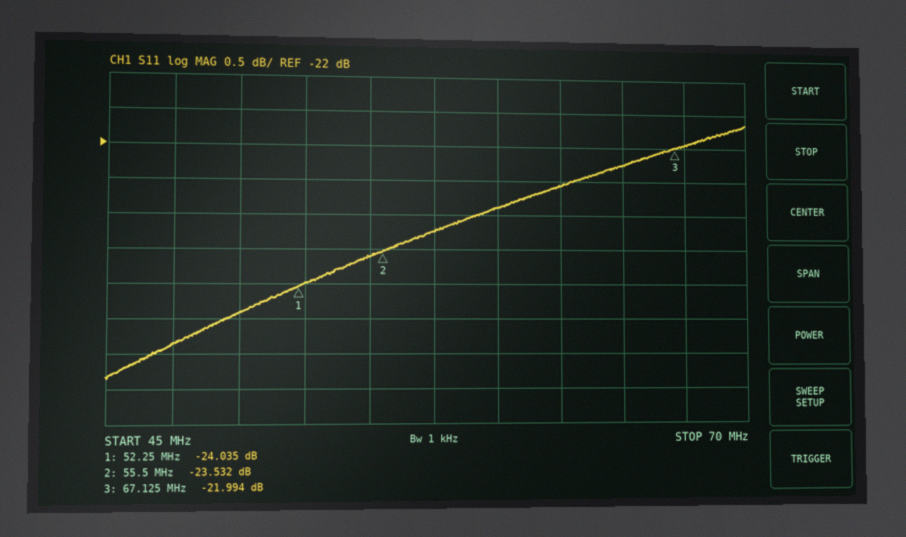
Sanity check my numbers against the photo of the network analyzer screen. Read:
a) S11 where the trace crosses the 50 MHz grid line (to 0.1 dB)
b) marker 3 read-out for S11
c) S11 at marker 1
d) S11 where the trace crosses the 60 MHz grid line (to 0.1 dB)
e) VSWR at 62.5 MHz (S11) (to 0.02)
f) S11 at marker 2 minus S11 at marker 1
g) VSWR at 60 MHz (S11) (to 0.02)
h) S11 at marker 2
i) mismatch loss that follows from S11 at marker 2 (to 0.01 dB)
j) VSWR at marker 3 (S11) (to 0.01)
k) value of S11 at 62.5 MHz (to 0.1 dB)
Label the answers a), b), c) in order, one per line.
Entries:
a) -24.4 dB
b) -21.994 dB
c) -24.035 dB
d) -22.9 dB
e) 1.16
f) 0.503 dB
g) 1.16
h) -23.532 dB
i) 0.02 dB
j) 1.17
k) -22.6 dB
